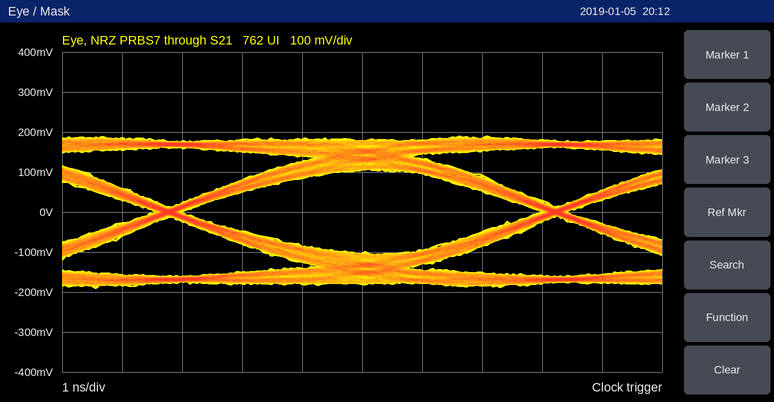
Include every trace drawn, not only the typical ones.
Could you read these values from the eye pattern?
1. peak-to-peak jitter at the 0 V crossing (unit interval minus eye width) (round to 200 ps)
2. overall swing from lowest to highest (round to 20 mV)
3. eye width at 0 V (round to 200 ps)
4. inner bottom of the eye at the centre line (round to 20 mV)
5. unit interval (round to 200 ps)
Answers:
400 ps
380 mV
6.0 ns
-100 mV
6.4 ns
